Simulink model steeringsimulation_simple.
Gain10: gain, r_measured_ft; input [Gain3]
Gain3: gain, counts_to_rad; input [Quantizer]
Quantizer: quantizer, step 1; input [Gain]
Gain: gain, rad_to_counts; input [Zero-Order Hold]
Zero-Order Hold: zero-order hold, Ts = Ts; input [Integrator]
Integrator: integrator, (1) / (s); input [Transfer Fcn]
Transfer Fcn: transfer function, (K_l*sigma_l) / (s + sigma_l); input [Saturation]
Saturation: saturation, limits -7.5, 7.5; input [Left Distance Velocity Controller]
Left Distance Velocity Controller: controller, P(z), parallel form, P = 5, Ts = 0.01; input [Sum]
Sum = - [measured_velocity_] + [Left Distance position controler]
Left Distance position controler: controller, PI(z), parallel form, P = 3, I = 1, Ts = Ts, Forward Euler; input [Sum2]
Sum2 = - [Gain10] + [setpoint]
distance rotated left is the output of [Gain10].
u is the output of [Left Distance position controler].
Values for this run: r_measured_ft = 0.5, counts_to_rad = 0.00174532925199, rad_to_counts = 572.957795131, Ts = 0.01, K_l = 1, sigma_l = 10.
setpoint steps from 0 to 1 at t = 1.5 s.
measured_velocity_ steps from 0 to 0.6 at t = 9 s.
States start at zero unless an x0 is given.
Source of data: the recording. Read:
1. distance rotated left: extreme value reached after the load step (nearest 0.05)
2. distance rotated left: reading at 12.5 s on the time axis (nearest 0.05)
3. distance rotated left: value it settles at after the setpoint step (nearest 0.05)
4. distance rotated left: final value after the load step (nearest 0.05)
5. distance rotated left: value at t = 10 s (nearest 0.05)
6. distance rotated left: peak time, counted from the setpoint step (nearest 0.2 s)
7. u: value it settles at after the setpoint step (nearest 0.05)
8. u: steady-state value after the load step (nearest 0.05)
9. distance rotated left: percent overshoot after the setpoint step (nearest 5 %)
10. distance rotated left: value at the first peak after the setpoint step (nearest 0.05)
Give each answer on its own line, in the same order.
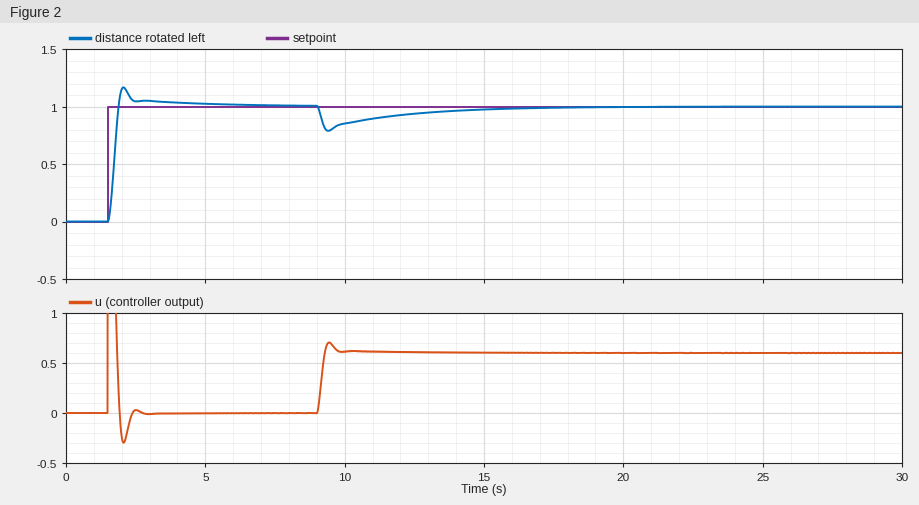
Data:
0.80
0.95
1.00
1.00
0.85
0.6 s
0.00
0.60
15 %
1.15
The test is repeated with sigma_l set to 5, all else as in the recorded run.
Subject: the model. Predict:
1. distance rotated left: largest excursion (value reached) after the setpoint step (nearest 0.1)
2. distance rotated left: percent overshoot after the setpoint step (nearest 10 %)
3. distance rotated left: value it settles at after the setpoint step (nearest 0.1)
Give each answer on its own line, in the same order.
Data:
1.3
30 %
1.0
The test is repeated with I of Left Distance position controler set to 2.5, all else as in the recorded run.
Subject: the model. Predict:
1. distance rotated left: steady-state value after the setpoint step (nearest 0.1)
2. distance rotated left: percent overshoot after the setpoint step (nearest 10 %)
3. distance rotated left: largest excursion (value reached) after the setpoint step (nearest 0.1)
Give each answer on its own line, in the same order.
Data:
1.0
30 %
1.3
